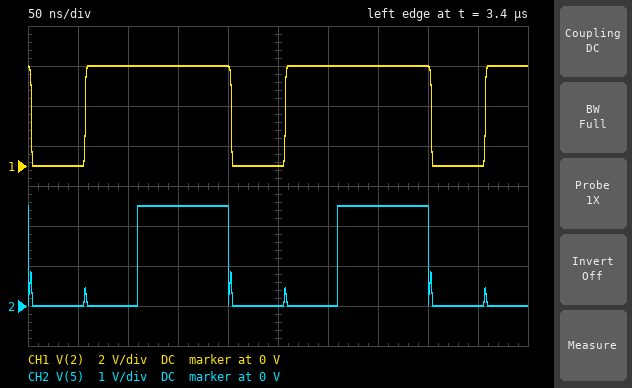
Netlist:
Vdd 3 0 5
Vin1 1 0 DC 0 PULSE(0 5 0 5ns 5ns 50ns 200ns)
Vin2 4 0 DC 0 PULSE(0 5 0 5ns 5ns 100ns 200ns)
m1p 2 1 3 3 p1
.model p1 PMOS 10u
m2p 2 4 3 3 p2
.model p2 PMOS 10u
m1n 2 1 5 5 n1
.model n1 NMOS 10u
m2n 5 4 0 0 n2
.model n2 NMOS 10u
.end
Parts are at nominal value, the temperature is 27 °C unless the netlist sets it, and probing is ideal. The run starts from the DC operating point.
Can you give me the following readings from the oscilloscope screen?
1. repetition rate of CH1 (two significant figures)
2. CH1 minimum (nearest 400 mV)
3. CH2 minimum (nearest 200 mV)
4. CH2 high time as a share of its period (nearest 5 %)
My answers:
5.0 MHz
0 V
0 V
45 %
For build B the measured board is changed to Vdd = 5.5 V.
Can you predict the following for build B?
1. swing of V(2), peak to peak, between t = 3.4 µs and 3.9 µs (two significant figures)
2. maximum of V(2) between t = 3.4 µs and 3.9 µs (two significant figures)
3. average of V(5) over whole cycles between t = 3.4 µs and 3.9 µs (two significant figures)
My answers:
5.4 V
5.5 V
1.3 V
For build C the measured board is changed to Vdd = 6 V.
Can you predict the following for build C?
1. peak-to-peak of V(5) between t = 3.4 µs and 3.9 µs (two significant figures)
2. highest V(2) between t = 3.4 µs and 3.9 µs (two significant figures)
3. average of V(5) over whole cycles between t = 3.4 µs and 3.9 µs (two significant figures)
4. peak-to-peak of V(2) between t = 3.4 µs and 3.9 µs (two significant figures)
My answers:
3.0 V
6.0 V
1.4 V
5.6 V
